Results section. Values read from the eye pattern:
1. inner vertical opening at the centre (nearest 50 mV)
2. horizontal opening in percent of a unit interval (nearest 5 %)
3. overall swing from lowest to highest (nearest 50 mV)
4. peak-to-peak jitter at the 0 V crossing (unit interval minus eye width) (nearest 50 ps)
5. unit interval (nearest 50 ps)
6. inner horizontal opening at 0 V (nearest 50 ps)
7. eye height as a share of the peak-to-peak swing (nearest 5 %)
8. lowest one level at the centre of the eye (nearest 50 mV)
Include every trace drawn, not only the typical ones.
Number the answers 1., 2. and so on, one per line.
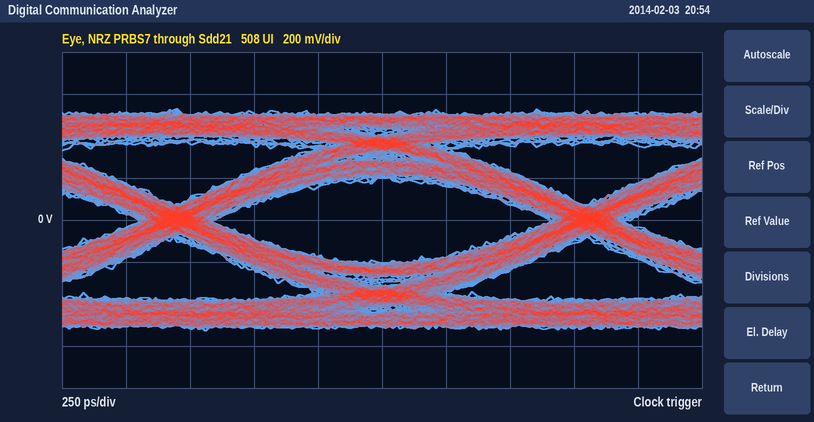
1. 400 mV
2. 80 %
3. 1.05 V
4. 300 ps
5. 1.60 ns
6. 1.30 ns
7. 40 %
8. 200 mV
